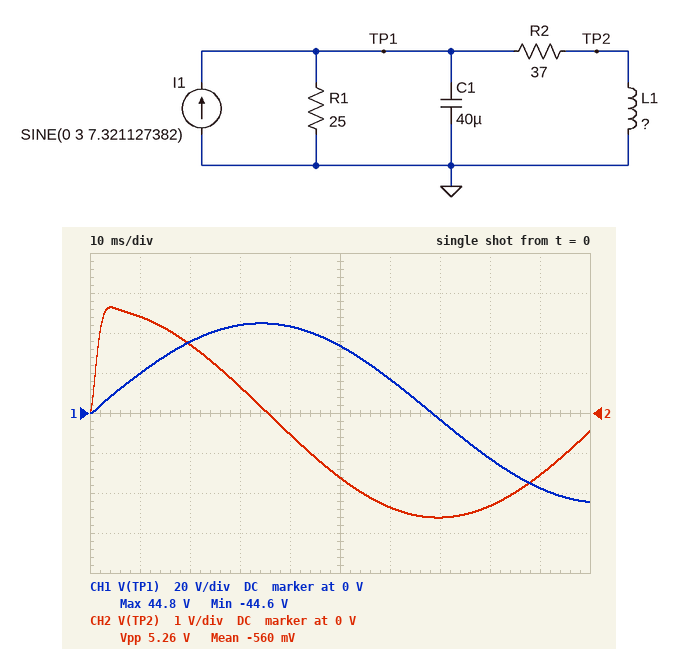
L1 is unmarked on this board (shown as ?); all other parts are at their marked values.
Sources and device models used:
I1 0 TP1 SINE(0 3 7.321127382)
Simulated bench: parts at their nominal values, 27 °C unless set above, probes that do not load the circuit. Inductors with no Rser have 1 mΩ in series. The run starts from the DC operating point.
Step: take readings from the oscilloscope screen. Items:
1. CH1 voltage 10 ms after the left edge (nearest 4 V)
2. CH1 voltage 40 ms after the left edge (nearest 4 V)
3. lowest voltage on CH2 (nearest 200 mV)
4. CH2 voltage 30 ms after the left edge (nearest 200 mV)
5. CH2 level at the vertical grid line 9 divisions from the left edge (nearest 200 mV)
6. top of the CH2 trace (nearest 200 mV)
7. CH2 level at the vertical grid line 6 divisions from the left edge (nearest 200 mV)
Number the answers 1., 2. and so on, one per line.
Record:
1. 20 V
2. 44 V
3. -2.6 V
4. 600 mV
5. -1.6 V
6. 2.6 V
7. -2.4 V
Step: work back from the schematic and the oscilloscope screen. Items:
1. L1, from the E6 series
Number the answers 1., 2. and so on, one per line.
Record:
1. 47 mH
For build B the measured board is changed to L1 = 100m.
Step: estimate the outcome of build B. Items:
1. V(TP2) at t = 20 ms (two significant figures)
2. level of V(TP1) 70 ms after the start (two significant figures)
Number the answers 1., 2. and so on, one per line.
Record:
1. 3.8 V
2. -4.5 V
